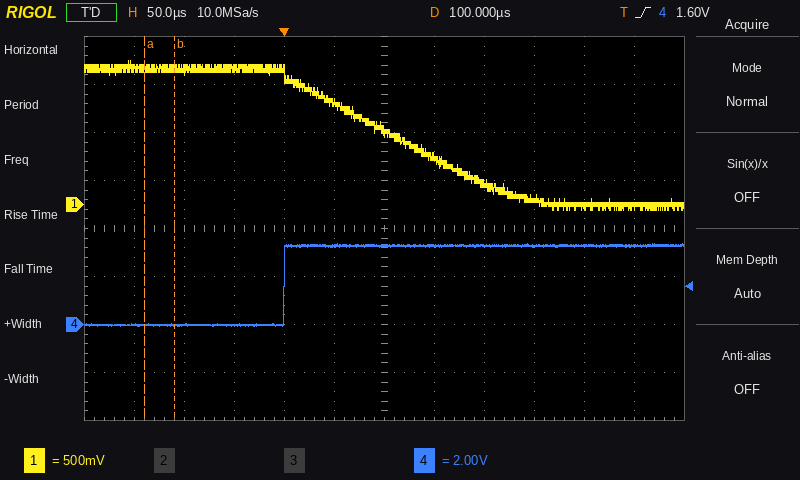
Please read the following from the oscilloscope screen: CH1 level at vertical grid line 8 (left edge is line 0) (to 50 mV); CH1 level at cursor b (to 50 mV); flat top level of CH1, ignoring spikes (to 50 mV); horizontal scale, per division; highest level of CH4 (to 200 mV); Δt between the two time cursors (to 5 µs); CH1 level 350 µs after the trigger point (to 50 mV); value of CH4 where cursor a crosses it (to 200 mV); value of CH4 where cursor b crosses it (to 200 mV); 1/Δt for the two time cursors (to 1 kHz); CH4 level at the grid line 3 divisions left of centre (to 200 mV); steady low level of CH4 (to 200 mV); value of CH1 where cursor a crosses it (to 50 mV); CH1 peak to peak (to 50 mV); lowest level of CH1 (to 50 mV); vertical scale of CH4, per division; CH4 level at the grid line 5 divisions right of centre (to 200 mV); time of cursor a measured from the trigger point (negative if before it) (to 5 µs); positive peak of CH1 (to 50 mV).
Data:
200 mV
1.40 V
1.40 V
50 µs
3.4 V
30 µs
0 mV
0.0 V
0.0 V
33 kHz
0.0 V
0.0 V
1.40 V
1.55 V
-50 mV
2 V
3.2 V
-140 µs
1.50 V
